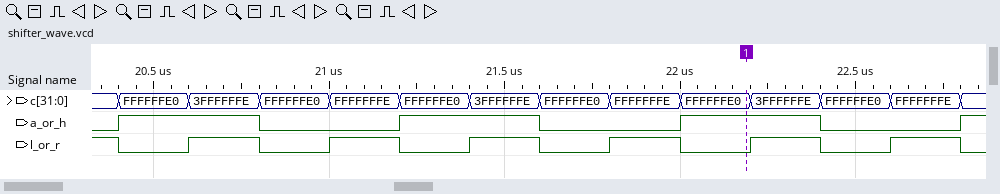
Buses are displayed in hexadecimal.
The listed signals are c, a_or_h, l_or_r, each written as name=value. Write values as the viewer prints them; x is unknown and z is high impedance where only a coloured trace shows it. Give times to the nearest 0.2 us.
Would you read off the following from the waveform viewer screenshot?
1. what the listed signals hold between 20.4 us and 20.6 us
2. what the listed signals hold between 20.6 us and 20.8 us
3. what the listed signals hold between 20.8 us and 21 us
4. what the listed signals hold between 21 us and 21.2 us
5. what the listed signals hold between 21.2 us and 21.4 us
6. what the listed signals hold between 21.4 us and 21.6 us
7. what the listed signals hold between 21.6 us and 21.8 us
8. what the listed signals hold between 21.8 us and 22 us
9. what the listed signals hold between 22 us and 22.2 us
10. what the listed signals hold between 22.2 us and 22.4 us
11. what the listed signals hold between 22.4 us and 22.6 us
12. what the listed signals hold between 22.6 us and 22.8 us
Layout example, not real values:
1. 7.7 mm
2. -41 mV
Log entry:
1. c=FFFFFFE0, a_or_h=1, l_or_r=0
2. c=3FFFFFFE, a_or_h=1, l_or_r=1
3. c=FFFFFFE0, a_or_h=0, l_or_r=0
4. c=FFFFFFFE, a_or_h=0, l_or_r=1
5. c=FFFFFFE0, a_or_h=1, l_or_r=0
6. c=3FFFFFFE, a_or_h=1, l_or_r=1
7. c=FFFFFFE0, a_or_h=0, l_or_r=0
8. c=FFFFFFFE, a_or_h=0, l_or_r=1
9. c=FFFFFFE0, a_or_h=1, l_or_r=0
10. c=3FFFFFFE, a_or_h=1, l_or_r=1
11. c=FFFFFFE0, a_or_h=0, l_or_r=0
12. c=FFFFFFFE, a_or_h=0, l_or_r=1
